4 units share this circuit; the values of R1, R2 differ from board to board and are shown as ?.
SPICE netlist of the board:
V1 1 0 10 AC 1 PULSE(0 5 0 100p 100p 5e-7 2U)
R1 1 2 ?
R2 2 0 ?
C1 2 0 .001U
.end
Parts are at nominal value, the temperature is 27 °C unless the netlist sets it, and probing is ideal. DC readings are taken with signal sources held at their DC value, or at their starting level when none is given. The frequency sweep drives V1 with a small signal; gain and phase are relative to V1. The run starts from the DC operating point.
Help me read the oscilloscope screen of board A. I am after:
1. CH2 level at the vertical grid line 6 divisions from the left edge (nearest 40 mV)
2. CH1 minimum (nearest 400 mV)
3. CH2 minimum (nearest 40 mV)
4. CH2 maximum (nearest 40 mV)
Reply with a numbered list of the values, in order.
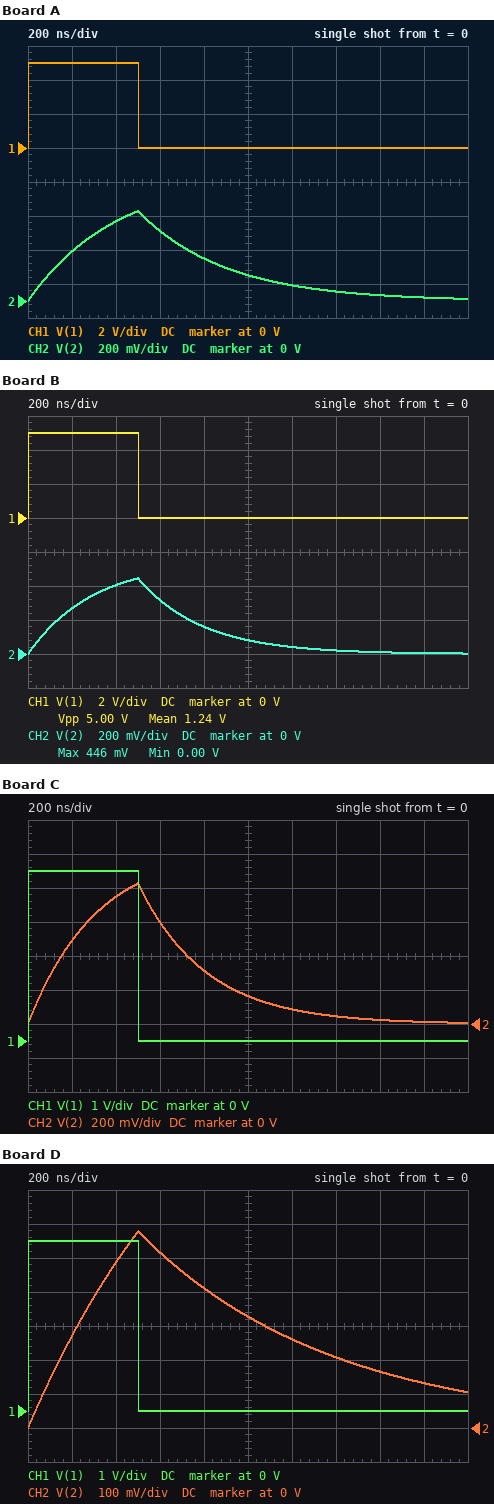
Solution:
1. 80 mV
2. 0 V
3. 0 V
4. 520 mV
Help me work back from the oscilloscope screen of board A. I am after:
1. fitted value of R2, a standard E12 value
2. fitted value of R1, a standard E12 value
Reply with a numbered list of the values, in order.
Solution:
1. 470 Ω
2. 2.7 kΩ
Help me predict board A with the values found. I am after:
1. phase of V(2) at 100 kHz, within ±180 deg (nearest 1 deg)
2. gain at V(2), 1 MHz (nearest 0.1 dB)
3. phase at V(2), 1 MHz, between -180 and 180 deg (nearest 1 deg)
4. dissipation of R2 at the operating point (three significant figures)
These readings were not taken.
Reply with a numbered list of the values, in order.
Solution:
1. -14 deg
2. -25.2 dB
3. -68 deg
4. 4.68 mW
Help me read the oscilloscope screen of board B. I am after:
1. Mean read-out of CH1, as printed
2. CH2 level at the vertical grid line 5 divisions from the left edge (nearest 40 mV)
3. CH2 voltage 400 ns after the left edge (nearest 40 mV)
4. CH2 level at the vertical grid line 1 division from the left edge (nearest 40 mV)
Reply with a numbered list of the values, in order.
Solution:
1. 1.24 V
2. 80 mV
3. 400 mV
4. 280 mV
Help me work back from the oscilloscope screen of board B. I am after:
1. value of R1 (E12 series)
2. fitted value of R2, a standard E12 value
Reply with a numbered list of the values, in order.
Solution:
1. 2.7 kΩ
2. 330 Ω
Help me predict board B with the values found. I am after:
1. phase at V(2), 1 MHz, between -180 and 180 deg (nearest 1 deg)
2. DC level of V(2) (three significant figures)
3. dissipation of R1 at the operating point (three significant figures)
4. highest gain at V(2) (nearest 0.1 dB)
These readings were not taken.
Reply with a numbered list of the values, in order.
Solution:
1. -62 deg
2. 1.09 V
3. 29.4 mW
4. -19.3 dB
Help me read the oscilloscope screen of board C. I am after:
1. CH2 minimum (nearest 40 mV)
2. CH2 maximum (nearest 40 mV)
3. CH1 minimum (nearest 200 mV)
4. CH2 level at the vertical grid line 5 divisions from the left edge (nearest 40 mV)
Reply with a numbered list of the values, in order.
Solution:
1. 0 V
2. 840 mV
3. 0 V
4. 160 mV
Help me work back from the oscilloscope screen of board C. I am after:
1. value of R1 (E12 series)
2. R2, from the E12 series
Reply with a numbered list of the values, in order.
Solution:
1. 1.5 kΩ
2. 390 Ω
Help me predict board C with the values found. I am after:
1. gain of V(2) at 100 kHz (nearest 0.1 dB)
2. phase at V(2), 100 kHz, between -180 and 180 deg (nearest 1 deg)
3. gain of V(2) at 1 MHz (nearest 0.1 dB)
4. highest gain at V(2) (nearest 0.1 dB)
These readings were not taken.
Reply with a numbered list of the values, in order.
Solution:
1. -13.9 dB
2. -11 deg
3. -20.5 dB
4. -13.7 dB
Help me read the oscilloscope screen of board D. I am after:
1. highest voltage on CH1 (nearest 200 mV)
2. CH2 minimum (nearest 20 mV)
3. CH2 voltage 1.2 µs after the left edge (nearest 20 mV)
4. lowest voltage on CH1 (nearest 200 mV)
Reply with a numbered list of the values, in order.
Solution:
1. 5.0 V
2. 0 V
3. 260 mV
4. 0 V
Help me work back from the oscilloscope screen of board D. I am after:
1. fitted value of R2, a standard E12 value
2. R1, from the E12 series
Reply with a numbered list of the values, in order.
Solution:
1. 1.2 kΩ
2. 3.3 kΩ
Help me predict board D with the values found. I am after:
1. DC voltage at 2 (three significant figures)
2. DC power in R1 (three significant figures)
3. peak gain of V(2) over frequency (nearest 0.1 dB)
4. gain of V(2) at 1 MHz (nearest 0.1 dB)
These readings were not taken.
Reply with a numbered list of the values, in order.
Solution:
1. 2.67 V
2. 16.3 mW
3. -11.5 dB
4. -26.5 dB
